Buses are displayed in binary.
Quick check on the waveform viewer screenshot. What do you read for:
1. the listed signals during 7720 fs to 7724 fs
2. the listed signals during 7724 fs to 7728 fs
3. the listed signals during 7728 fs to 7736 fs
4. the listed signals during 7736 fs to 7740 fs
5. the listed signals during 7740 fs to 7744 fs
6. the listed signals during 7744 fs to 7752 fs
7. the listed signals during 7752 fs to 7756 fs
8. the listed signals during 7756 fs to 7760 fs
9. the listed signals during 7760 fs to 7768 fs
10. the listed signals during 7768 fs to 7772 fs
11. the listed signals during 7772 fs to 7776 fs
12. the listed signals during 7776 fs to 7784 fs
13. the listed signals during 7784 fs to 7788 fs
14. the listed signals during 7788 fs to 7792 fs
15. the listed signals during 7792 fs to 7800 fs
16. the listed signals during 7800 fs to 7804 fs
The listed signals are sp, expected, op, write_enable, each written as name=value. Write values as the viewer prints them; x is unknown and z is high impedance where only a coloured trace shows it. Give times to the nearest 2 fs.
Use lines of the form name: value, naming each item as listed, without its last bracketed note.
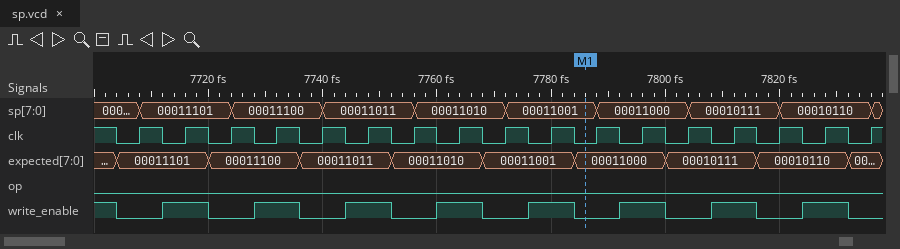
the listed signals during 7720 fs to 7724 fs: sp=00011101, expected=00011100, op=0, write_enable=0
the listed signals during 7724 fs to 7728 fs: sp=00011100, expected=00011100, op=0, write_enable=0
the listed signals during 7728 fs to 7736 fs: sp=00011100, expected=00011100, op=0, write_enable=1
the listed signals during 7736 fs to 7740 fs: sp=00011100, expected=00011011, op=0, write_enable=0
the listed signals during 7740 fs to 7744 fs: sp=00011011, expected=00011011, op=0, write_enable=0
the listed signals during 7744 fs to 7752 fs: sp=00011011, expected=00011011, op=0, write_enable=1
the listed signals during 7752 fs to 7756 fs: sp=00011011, expected=00011010, op=0, write_enable=0
the listed signals during 7756 fs to 7760 fs: sp=00011010, expected=00011010, op=0, write_enable=0
the listed signals during 7760 fs to 7768 fs: sp=00011010, expected=00011010, op=0, write_enable=1
the listed signals during 7768 fs to 7772 fs: sp=00011010, expected=00011001, op=0, write_enable=0
the listed signals during 7772 fs to 7776 fs: sp=00011001, expected=00011001, op=0, write_enable=0
the listed signals during 7776 fs to 7784 fs: sp=00011001, expected=00011001, op=0, write_enable=1
the listed signals during 7784 fs to 7788 fs: sp=00011001, expected=00011000, op=0, write_enable=0
the listed signals during 7788 fs to 7792 fs: sp=00011000, expected=00011000, op=0, write_enable=0
the listed signals during 7792 fs to 7800 fs: sp=00011000, expected=00011000, op=0, write_enable=1
the listed signals during 7800 fs to 7804 fs: sp=00011000, expected=00010111, op=0, write_enable=0
